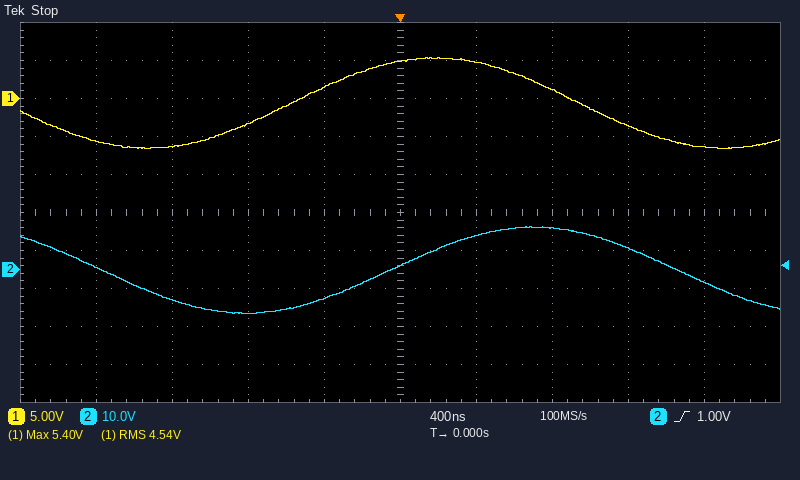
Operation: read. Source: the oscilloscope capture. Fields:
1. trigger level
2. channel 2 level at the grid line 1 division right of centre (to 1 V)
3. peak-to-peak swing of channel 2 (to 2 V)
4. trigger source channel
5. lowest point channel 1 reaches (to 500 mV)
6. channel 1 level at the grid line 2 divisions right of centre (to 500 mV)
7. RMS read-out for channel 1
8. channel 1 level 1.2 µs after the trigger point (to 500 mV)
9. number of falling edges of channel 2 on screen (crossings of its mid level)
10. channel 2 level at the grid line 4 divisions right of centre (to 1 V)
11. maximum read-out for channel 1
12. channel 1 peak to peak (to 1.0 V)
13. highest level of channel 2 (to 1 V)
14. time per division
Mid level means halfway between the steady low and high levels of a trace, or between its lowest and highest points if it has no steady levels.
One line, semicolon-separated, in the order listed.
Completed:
1.00 V; 9 V; 22 V; channel 2; -6.5 V; 1.0 V; 4.54 V; -3.5 V; 2; -3 V; 5.40 V; 12.0 V; 11 V; 400 ns
